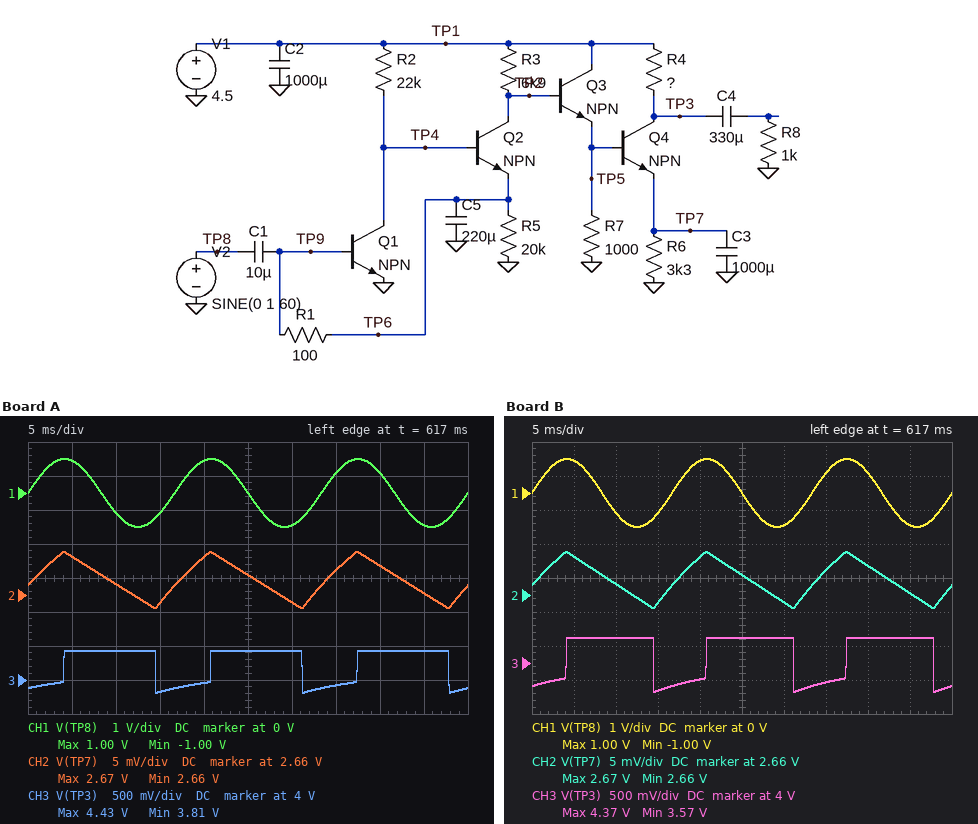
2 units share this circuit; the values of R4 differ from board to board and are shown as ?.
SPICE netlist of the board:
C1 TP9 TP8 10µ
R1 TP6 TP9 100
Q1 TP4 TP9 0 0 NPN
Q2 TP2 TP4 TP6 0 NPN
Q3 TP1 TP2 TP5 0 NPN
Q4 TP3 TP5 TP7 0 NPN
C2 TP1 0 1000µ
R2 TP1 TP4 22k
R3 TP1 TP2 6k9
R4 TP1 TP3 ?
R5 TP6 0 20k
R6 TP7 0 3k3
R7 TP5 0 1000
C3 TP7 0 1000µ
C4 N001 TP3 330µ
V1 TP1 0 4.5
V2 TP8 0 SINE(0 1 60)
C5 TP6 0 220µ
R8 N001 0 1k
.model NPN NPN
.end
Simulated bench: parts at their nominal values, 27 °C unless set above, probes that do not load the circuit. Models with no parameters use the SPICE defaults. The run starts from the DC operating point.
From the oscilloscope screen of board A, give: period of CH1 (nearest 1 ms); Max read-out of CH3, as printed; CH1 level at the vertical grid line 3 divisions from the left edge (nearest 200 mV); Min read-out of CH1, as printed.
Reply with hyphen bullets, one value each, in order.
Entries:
- 17 ms
- 4.43 V
- -600 mV
- -1.00 V
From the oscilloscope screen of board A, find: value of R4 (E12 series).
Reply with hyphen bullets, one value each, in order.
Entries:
- 330 Ω
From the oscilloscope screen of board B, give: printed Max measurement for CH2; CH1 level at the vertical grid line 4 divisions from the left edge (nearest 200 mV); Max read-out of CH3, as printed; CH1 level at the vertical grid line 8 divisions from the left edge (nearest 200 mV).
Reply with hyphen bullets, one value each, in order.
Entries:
- 2.67 V
- 1.0 V
- 4.37 V
- 600 mV
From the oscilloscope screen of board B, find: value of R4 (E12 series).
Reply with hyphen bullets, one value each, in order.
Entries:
- 470 Ω
